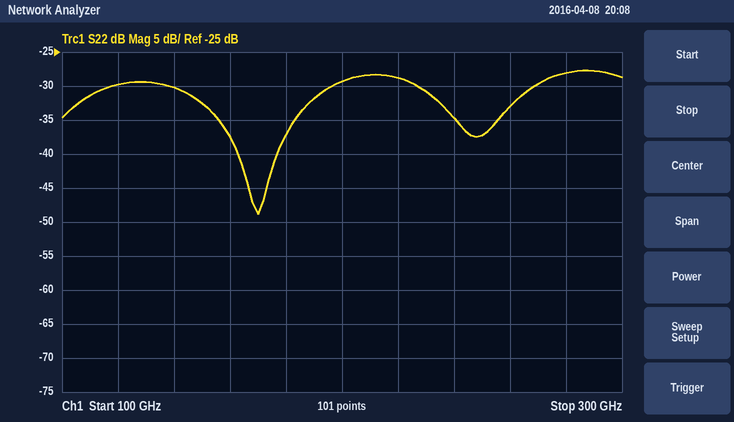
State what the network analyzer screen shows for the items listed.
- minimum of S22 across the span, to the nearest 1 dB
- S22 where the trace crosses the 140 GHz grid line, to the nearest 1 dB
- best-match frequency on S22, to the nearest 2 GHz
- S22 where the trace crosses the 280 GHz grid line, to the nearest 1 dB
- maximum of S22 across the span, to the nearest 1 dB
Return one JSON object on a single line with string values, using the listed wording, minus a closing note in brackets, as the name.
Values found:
{"minimum of S22 across the span, to the nearest 1 dB": "-49 dB", "S22 where the trace crosses the 140 GHz grid line, to the nearest 1 dB": "-30 dB", "best-match frequency on S22, to the nearest 2 GHz": "170 GHz", "S22 where the trace crosses the 280 GHz grid line, to the nearest 1 dB": "-28 dB", "maximum of S22 across the span, to the nearest 1 dB": "-28 dB"}
